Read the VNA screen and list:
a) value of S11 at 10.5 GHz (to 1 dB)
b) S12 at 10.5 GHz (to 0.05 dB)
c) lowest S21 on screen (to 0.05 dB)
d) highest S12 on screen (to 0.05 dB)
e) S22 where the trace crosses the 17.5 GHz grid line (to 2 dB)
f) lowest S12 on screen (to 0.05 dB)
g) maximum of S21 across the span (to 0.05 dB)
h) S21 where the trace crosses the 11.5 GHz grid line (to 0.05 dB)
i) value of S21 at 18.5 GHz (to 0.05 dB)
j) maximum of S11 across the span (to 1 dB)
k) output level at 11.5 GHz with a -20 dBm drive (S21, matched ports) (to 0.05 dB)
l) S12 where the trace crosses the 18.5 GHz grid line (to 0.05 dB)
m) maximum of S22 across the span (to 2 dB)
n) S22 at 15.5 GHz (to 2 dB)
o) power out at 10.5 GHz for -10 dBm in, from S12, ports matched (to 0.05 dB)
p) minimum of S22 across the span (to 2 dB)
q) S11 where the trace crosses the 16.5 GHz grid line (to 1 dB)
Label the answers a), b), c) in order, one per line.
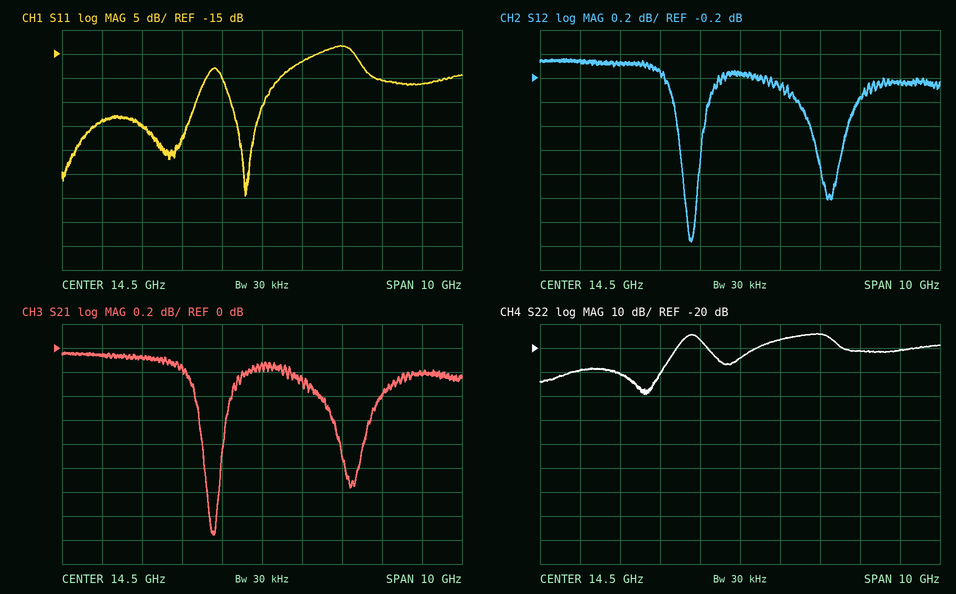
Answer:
a) -29 dB
b) -0.05 dB
c) -1.55 dB
d) -0.05 dB
e) -22 dB
f) -1.55 dB
g) -0.05 dB
h) -0.10 dB
i) -0.20 dB
j) -13 dB
k) -20.10 dBm
l) -0.25 dB
m) -14 dB
n) -16 dB
o) -10.05 dBm
p) -40 dB
q) -13 dB
